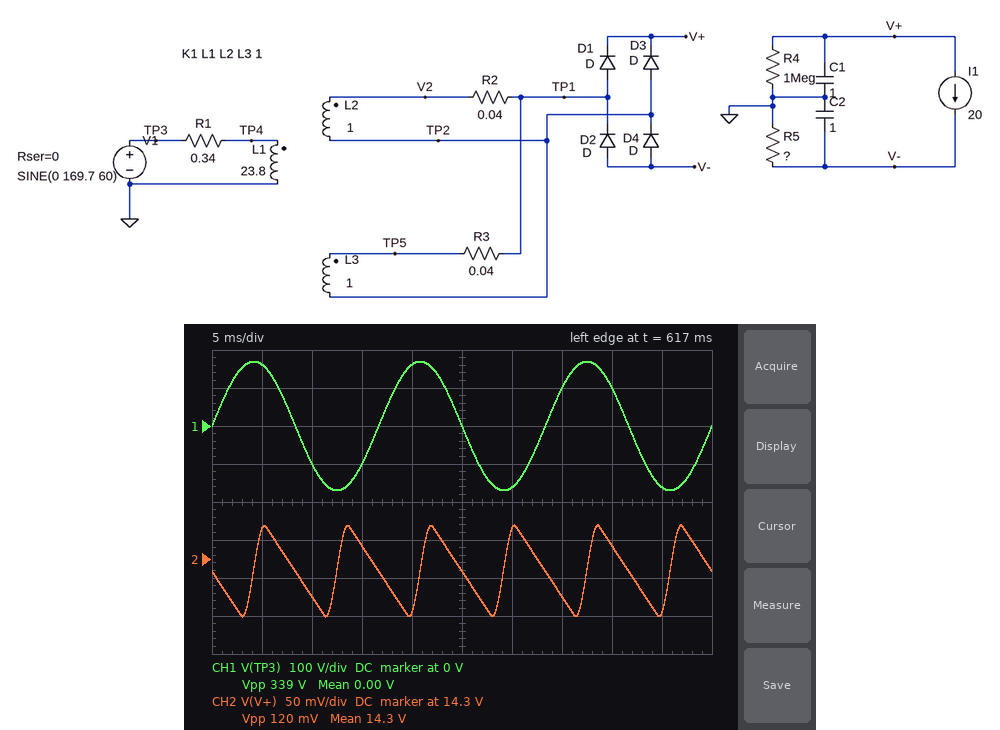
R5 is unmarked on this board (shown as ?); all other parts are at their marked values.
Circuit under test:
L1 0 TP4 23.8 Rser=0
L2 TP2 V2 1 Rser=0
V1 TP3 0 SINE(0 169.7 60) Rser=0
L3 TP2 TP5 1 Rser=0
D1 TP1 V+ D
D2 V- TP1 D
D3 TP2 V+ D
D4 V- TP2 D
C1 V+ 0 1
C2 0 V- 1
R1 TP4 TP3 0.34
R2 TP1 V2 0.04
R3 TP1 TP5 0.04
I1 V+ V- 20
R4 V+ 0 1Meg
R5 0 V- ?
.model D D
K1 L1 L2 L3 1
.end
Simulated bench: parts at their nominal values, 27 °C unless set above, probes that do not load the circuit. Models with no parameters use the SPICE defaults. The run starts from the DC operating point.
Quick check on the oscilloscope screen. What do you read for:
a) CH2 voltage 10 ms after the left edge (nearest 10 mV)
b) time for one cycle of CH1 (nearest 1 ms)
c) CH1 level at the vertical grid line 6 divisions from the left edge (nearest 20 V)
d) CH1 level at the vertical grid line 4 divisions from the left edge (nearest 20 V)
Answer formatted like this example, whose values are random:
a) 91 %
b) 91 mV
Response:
a) 14.25 V
b) 17 ms
c) -160 V
d) 160 V
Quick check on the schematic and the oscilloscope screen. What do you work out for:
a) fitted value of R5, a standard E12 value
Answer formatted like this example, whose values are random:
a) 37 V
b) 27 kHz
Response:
a) 390 kΩ
